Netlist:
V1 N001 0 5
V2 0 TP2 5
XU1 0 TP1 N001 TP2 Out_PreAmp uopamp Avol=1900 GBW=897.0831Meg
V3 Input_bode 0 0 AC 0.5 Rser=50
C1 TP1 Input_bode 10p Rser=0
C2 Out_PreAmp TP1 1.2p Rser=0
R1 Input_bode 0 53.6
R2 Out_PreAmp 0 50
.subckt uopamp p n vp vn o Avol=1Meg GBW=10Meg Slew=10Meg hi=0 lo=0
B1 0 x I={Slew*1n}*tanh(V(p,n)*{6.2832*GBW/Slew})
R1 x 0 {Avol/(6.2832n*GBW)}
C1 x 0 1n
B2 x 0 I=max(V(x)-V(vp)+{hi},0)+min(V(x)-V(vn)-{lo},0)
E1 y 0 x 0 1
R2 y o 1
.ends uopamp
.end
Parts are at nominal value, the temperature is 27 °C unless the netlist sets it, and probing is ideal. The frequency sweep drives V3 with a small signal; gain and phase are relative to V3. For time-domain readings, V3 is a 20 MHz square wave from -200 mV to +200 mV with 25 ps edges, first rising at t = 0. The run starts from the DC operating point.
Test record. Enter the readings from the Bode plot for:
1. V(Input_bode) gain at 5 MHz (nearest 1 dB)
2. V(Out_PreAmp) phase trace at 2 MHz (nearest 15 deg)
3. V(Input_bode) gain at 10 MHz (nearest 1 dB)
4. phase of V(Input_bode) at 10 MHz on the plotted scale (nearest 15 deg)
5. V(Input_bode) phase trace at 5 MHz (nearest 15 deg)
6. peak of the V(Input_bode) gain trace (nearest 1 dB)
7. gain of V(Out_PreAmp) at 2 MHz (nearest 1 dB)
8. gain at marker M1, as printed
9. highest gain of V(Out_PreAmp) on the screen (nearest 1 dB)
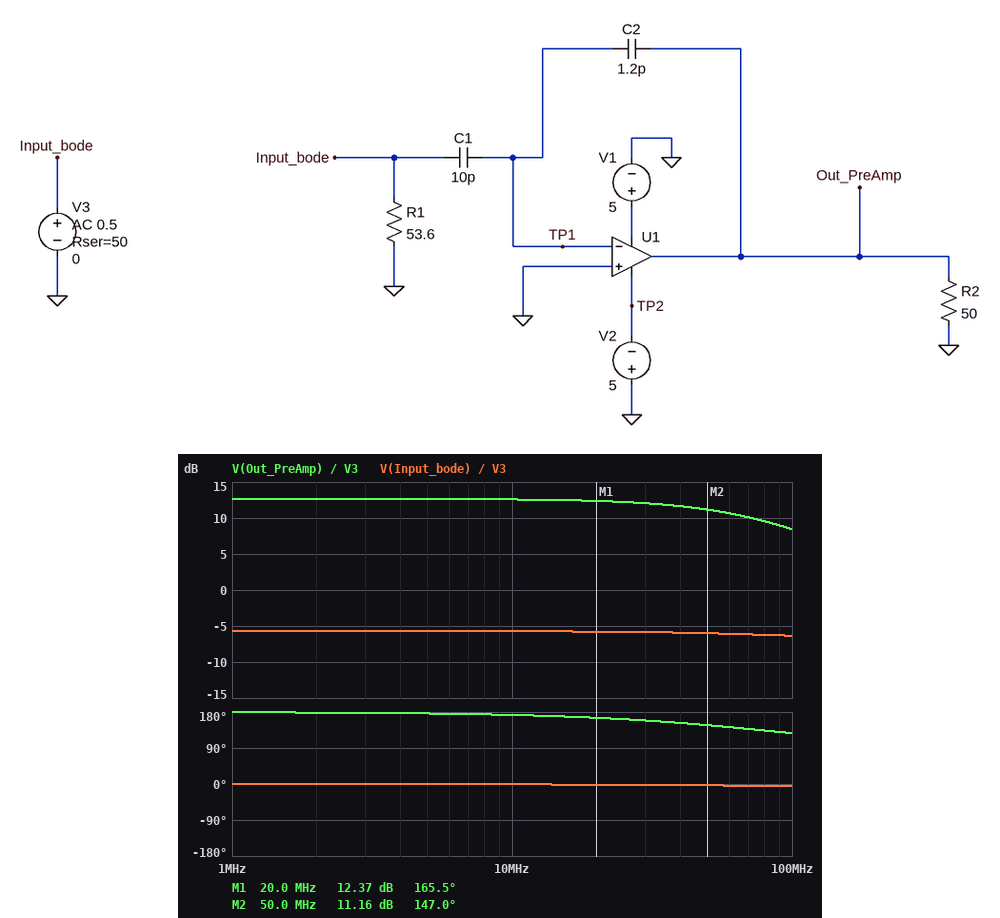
-6 dB
180 deg
-6 dB
0 deg
0 deg
-6 dB
13 dB
12.37 dB
13 dB
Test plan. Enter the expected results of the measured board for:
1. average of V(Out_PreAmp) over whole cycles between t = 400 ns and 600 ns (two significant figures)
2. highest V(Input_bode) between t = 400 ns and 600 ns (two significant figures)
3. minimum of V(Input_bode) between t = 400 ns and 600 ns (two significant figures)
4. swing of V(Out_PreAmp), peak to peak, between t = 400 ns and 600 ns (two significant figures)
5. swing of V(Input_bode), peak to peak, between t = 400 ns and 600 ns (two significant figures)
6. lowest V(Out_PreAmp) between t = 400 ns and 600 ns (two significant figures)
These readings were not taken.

-120 mV
100 mV
-100 mV
250 mV
210 mV
-250 mV
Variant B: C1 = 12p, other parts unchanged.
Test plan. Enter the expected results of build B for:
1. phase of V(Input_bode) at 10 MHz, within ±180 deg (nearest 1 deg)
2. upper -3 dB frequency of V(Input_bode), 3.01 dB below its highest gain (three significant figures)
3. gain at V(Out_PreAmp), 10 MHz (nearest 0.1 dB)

-1 deg
4.52 GHz
14.1 dB
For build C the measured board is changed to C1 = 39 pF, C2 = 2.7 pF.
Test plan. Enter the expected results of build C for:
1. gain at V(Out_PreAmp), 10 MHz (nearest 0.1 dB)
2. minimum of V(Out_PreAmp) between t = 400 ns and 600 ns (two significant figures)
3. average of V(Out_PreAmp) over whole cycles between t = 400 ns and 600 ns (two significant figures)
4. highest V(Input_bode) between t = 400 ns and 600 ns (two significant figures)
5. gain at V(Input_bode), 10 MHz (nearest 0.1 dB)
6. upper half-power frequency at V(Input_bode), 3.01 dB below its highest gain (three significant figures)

17.2 dB
-260 mV
-130 mV
100 mV
-5.8 dB
1.04 GHz
